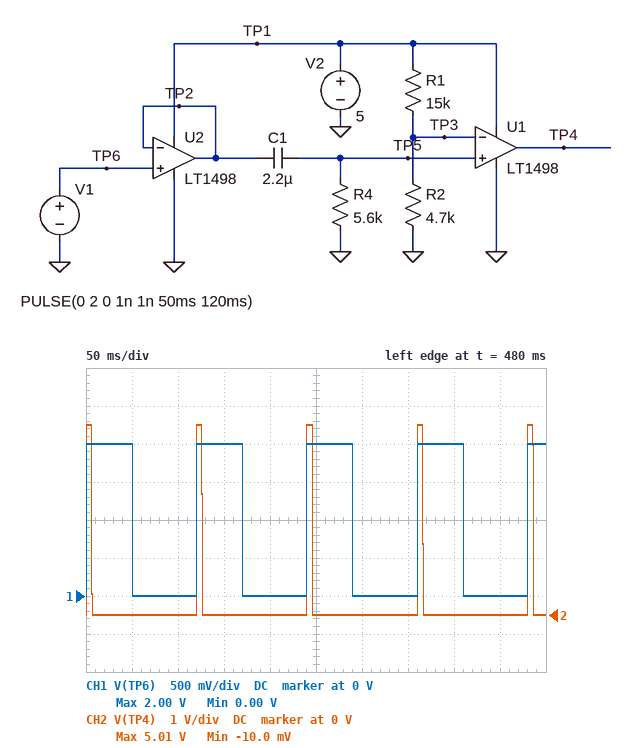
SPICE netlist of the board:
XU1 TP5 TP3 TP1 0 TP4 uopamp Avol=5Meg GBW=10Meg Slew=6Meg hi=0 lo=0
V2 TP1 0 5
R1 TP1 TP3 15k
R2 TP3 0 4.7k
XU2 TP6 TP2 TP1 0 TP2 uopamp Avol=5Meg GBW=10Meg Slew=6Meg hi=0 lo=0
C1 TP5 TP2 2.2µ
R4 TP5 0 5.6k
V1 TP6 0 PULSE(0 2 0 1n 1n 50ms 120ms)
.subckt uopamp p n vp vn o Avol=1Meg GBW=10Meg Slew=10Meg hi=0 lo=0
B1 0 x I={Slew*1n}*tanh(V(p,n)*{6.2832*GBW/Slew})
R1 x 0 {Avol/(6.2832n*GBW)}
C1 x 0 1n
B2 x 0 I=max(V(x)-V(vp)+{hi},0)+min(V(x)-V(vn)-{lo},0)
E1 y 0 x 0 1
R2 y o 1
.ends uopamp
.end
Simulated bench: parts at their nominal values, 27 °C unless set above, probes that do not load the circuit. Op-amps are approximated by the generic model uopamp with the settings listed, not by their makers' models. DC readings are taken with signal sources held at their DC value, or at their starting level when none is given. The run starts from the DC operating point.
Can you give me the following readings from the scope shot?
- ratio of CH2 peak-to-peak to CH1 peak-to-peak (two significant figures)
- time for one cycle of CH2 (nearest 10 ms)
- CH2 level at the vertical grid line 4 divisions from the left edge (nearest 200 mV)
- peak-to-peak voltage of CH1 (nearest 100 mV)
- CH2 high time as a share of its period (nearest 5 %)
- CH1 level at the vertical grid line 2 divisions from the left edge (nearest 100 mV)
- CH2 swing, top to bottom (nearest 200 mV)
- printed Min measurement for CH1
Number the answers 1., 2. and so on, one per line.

1. 2.5
2. 120 ms
3. 0 V
4. 2.0 V
5. 5 %
6. 0 V
7. 5.0 V
8. 0.00 V
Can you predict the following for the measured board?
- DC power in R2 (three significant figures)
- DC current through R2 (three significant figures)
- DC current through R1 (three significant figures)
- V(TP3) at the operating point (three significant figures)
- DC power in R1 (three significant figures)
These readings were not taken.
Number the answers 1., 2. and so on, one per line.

1. 303 µW
2. 254 µA
3. 254 µA
4. 1.19 V
5. 966 µW
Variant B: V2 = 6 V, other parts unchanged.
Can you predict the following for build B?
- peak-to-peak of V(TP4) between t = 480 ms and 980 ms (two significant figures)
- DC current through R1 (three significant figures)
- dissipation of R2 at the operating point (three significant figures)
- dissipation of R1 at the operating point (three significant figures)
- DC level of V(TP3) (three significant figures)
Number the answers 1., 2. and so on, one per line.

1. 6.0 V
2. 305 µA
3. 436 µW
4. 1.39 mW
5. 1.43 V
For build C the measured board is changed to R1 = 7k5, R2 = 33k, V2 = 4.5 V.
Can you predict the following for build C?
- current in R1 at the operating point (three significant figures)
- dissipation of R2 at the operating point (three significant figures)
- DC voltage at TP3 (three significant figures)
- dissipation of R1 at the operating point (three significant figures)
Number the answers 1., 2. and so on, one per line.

1. 111 µA
2. 407 µW
3. 3.67 V
4. 92.6 µW
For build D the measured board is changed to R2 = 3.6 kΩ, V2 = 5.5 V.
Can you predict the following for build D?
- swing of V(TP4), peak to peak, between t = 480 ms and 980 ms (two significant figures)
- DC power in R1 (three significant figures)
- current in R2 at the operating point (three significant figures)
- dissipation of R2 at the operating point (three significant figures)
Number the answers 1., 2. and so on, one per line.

1. 5.5 V
2. 1.31 mW
3. 296 µA
4. 315 µW
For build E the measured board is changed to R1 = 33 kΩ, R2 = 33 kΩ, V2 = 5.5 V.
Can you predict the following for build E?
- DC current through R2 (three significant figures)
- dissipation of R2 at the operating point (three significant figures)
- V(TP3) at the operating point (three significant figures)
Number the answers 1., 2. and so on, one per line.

1. 83.3 µA
2. 229 µW
3. 2.75 V
